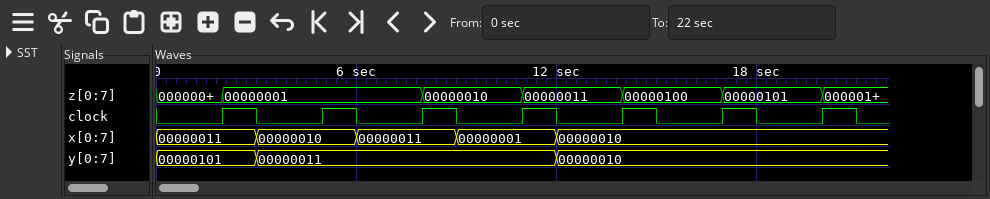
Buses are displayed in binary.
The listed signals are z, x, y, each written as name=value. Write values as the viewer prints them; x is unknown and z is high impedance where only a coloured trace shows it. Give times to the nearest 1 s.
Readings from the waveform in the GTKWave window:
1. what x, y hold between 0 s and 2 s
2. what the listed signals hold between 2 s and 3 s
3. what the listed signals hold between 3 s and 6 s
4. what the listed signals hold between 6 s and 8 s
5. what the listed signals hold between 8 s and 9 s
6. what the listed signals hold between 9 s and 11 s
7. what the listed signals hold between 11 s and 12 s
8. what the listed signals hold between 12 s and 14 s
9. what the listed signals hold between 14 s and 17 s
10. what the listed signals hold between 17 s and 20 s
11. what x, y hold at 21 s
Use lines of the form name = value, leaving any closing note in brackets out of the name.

what x, y hold between 0 s and 2 s = x=00000011, y=00000101
what the listed signals hold between 2 s and 3 s = z=00000001, x=00000011, y=00000101
what the listed signals hold between 3 s and 6 s = z=00000001, x=00000010, y=00000011
what the listed signals hold between 6 s and 8 s = z=00000001, x=00000011, y=00000011
what the listed signals hold between 8 s and 9 s = z=00000010, x=00000011, y=00000011
what the listed signals hold between 9 s and 11 s = z=00000010, x=00000001, y=00000011
what the listed signals hold between 11 s and 12 s = z=00000011, x=00000001, y=00000011
what the listed signals hold between 12 s and 14 s = z=00000011, x=00000010, y=00000010
what the listed signals hold between 14 s and 17 s = z=00000100, x=00000010, y=00000010
what the listed signals hold between 17 s and 20 s = z=00000101, x=00000010, y=00000010
what x, y hold at 21 s = x=00000010, y=00000010
